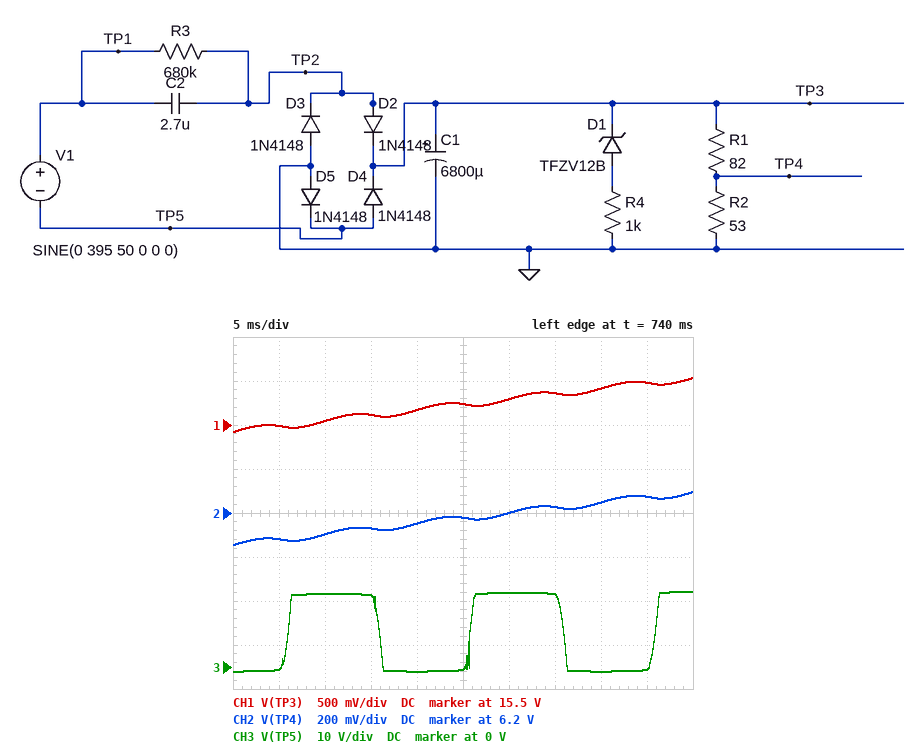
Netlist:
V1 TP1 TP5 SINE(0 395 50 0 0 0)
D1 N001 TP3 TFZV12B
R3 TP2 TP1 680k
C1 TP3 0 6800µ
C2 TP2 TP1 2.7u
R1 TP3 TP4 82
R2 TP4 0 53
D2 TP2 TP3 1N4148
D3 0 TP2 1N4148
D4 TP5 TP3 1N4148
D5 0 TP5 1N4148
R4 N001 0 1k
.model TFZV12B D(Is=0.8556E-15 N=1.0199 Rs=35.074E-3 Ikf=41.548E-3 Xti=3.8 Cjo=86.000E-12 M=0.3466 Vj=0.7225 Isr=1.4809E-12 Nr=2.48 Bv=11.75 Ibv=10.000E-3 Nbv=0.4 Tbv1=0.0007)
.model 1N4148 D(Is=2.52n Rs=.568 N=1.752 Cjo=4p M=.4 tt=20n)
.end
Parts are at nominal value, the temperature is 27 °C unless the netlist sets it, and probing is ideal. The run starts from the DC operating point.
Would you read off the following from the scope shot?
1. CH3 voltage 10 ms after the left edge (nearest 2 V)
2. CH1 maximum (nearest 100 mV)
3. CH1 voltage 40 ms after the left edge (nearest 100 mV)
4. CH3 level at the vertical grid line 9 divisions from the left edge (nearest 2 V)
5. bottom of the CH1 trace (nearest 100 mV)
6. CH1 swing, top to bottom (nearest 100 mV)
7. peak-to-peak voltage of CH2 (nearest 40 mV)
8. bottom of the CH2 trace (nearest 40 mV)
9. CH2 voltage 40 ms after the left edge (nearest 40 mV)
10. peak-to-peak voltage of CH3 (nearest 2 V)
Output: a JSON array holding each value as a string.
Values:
["16 V", "16.0 V", "15.9 V", "0 V", "15.4 V", "600 mV", "240 mV", "6.04 V", "6.24 V", "18 V"]
